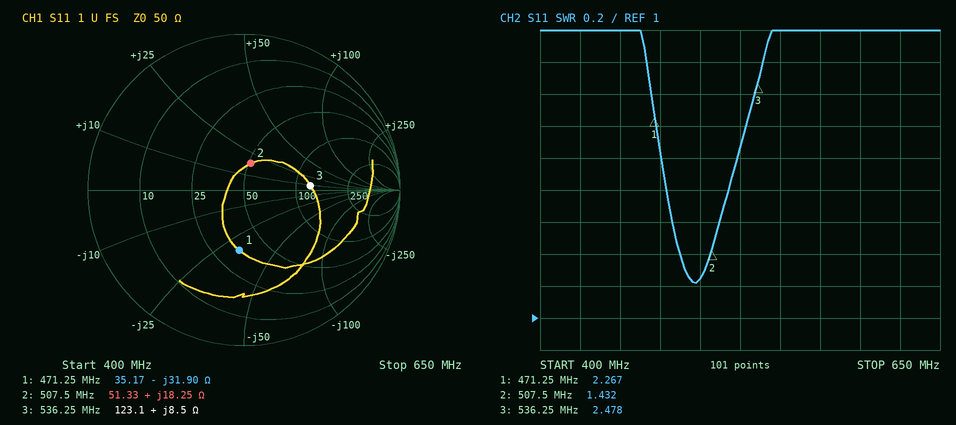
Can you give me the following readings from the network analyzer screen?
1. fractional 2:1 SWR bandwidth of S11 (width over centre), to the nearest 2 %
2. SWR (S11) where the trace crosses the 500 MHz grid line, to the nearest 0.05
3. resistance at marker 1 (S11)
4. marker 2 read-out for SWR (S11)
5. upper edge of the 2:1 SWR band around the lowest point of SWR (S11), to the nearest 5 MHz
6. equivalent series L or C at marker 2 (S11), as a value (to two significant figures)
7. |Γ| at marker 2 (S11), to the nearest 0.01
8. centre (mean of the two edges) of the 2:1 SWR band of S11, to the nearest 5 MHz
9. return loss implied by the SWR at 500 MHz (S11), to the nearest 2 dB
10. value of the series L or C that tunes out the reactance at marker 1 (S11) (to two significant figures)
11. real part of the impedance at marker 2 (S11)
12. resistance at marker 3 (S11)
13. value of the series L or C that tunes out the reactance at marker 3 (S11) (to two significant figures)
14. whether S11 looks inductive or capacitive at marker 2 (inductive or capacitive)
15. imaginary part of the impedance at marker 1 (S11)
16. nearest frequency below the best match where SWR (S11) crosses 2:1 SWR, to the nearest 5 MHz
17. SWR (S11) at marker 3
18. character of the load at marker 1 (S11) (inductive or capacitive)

10 %
1.25
35.17 Ω
1.432
525 MHz
5.7 nH
0.18
500 MHz
20 dB
11 nH
51.33 Ω
123.1 Ω
35 pF
inductive
-31.90 Ω
475 MHz
2.478
capacitive
